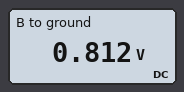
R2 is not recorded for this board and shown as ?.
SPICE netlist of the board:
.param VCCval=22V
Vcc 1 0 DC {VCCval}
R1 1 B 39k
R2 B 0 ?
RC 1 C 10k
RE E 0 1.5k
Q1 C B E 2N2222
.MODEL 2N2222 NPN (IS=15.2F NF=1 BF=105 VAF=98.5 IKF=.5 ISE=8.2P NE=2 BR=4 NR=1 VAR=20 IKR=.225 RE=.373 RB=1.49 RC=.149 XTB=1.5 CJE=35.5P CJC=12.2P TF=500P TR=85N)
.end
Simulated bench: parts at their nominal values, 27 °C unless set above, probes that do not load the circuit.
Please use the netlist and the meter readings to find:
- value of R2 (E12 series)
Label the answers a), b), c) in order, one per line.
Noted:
a) 1.5 kΩ
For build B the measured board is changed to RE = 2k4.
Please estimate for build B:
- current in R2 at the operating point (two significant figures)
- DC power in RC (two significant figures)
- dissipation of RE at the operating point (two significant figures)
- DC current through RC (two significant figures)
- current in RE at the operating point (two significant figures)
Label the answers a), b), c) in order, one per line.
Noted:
a) 540 µA
b) 92 µW
c) 23 µW
d) 96 µA
e) 97 µA
